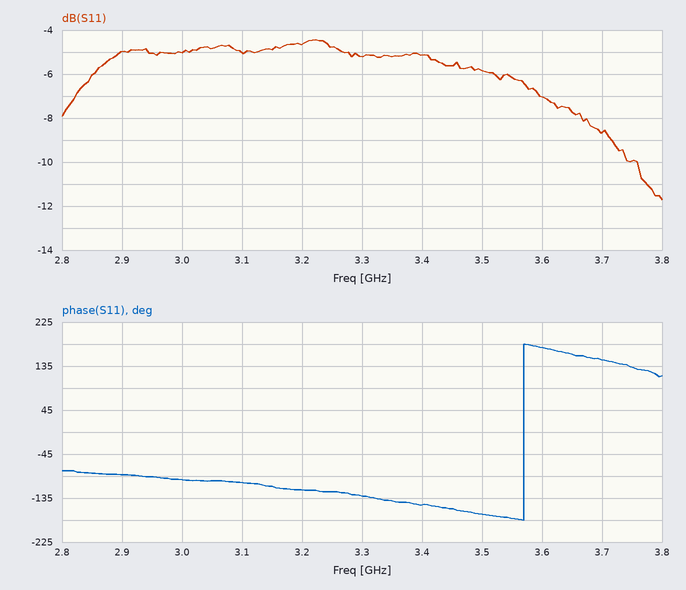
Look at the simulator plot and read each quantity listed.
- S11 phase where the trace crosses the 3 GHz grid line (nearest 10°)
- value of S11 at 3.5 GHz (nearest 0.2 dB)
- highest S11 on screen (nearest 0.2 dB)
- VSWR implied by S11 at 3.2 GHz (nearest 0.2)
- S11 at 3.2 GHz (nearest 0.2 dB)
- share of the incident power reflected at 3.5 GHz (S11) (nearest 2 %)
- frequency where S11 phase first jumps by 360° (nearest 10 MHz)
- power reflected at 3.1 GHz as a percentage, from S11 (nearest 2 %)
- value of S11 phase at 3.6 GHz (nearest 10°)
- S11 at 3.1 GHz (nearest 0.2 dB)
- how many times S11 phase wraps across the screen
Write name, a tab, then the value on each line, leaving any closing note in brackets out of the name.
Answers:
S11 phase where the trace crosses the 3 GHz grid line	-100°
value of S11 at 3.5 GHz	-5.8 dB
highest S11 on screen	-4.4 dB
VSWR implied by S11 at 3.2 GHz	3.8
S11 at 3.2 GHz	-4.6 dB
share of the incident power reflected at 3.5 GHz (S11)	26 %
frequency where S11 phase first jumps by 360°	3.57 GHz
power reflected at 3.1 GHz as a percentage, from S11	32 %
value of S11 phase at 3.6 GHz	170°
S11 at 3.1 GHz	-5.0 dB
how many times S11 phase wraps across the screen	1
